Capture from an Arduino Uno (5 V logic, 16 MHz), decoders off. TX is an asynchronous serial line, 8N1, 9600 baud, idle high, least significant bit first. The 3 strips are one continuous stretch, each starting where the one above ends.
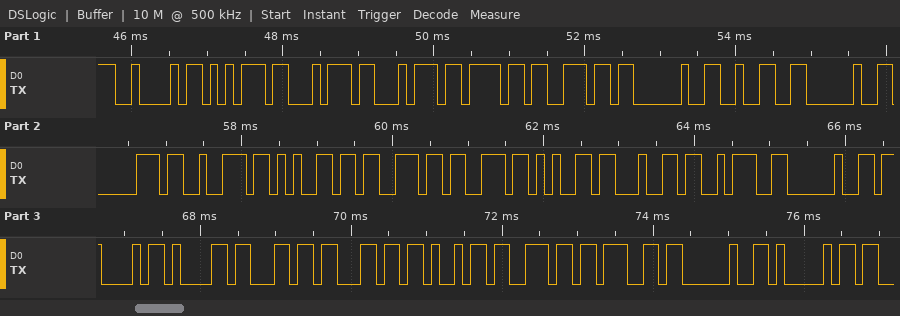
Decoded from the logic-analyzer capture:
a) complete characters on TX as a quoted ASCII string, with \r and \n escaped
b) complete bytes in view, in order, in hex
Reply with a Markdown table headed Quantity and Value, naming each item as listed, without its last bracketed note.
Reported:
| Quantity | Value |
|---|---|
| complete characters on TX as a quoted ASCII string, with \r and \n escaped | "Button 2 pressed: Calling A" |
| complete bytes in view, in order, in hex | 42 75 74 74 6F 6E 20 32 20 70 72 65 73 73 65 64 3A 20 43 61 6C 6C 69 6E 67 20 41 |
